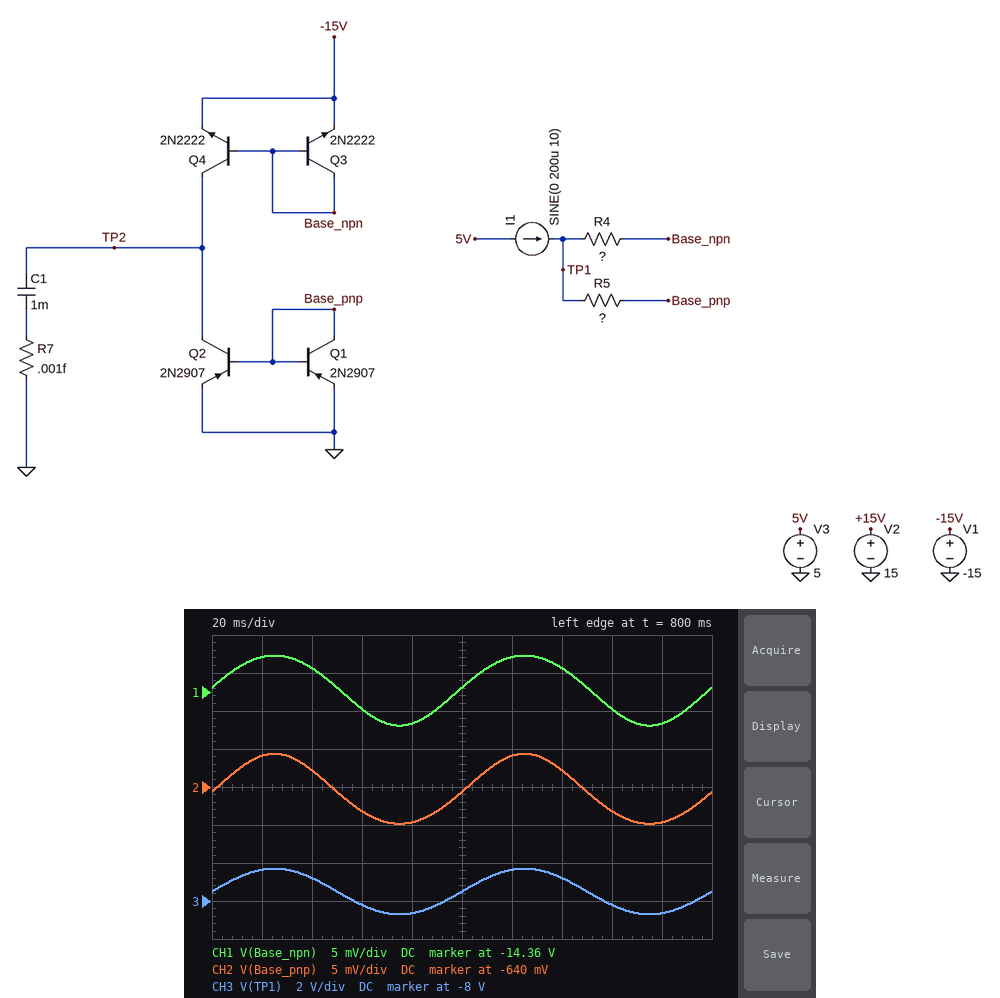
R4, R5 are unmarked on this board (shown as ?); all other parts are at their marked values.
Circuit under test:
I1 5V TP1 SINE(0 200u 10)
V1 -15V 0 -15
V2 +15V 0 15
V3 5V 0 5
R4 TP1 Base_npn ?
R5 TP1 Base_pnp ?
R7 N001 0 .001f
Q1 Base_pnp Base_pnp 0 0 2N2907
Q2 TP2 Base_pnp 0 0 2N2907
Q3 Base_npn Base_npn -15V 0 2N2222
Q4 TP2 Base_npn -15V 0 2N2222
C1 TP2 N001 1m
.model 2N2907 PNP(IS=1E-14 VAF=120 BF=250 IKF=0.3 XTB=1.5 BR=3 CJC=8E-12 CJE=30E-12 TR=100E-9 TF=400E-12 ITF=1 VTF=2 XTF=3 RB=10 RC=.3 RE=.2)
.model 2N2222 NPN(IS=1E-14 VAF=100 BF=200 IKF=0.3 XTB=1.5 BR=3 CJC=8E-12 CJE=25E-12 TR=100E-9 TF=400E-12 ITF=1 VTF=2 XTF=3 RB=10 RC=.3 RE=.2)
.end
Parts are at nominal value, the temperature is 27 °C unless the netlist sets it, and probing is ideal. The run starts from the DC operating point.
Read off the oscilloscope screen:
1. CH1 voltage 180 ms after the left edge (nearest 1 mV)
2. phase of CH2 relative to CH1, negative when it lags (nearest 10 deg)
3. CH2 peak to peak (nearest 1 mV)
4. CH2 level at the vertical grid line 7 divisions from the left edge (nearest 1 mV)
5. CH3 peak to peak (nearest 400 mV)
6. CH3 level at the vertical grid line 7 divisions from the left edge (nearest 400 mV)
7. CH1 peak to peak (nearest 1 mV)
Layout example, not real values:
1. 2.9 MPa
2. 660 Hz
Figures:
1. -14.364 V
2. 0 deg
3. 9 mV
4. -638 mV
5. 2.4 V
6. -6.8 V
7. 9 mV
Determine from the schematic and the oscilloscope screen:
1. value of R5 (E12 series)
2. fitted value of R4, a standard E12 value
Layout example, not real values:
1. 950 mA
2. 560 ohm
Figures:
1. 12 kΩ
2. 12 kΩ
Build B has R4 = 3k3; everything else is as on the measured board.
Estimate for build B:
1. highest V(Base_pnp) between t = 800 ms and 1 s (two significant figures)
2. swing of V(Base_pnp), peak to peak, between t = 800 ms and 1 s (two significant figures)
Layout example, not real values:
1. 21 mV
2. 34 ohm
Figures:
1. -650 mV
2. 2.5 mV
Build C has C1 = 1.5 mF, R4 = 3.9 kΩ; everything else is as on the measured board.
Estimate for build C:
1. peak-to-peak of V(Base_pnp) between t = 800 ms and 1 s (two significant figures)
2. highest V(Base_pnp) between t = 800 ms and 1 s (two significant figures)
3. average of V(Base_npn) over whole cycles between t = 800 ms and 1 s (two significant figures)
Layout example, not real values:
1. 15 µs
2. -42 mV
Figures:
1. 3.0 mV
2. -650 mV
3. -14 V
